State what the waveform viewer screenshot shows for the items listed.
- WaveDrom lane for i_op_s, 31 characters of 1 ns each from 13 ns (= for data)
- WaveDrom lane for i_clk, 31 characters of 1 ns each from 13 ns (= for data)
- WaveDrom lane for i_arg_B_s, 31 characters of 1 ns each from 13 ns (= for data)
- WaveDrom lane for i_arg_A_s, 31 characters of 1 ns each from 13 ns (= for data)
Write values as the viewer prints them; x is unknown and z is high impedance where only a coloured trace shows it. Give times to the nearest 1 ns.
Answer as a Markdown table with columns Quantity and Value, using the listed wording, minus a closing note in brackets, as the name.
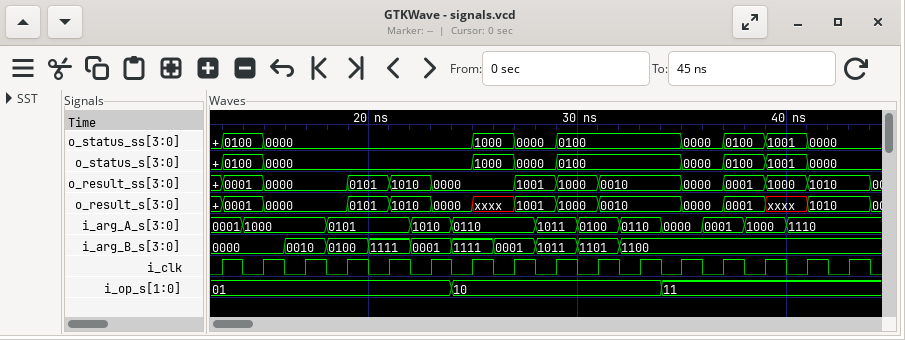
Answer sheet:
| Quantity | Value |
|---|---|
| WaveDrom lane for i_op_s, 31 characters of 1 ns each from 13 ns | {name: 'i_op_s', wave: '=..........=.........=.........', data: '01 10 11'} |
| WaveDrom lane for i_clk, 31 characters of 1 ns each from 13 ns | {name: 'i_clk', wave: '1010101010101010101010101010101'} |
| WaveDrom lane for i_arg_B_s, 31 characters of 1 ns each from 13 ns | {name: 'i_arg_B_s', wave: '=..=.=.=.=.=.=.=.=.=...........', data: '0000 0010 0100 1111 0001 1111 0001 1011 1101 1100'} |
| WaveDrom lane for i_arg_A_s, 31 characters of 1 ns each from 13 ns | {name: 'i_arg_A_s', wave: '==...=...=.=...=.=.=.=.=.=.=...', data: '0001 1000 0101 1010 0110 1011 0100 0110 0000 0001 1000 1110'} |
